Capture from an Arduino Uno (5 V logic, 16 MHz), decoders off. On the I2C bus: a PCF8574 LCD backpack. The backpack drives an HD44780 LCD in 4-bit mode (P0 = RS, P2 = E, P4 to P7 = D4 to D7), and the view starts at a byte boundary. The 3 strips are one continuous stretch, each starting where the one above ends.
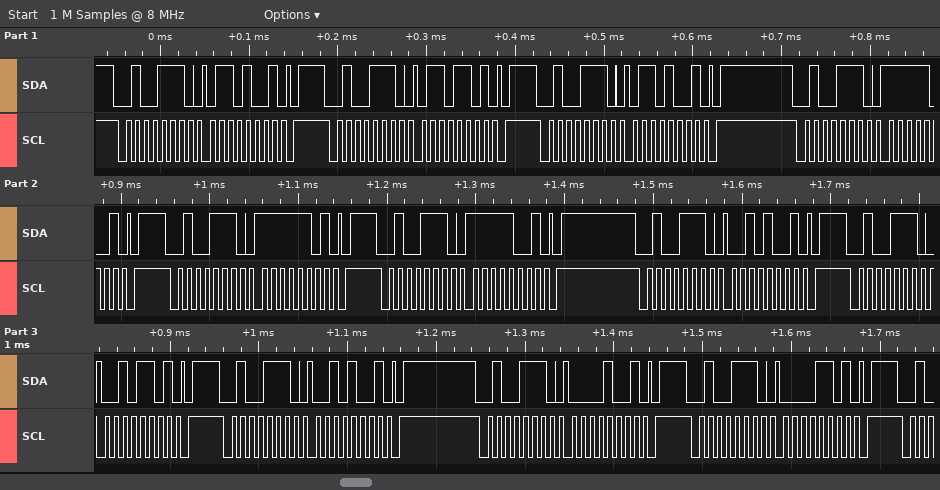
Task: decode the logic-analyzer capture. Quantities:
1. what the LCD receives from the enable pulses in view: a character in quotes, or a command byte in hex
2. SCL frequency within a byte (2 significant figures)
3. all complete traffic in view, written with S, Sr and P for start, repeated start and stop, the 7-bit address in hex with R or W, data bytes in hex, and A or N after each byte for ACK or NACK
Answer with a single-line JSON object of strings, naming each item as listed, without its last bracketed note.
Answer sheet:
{"what the LCD receives from the enable pulses in view: a character in quotes, or a command byte in hex": "'o'", "SCL frequency within a byte": "100 kHz", "all complete traffic in view, written with S, Sr and P for start, repeated start and stop, the 7-bit address in hex with R or W, data bytes in hex, and A or N after each byte for ACK or NACK": "S 27W A 69 A P S 27W A 6D A P S 27W A 69 A P S 27W A F9 A P S 27W A FD A P S 27W A F9 A P S 27W A 29 A P S 27W A 2D A P S 27W A 29 A P S 27W A 09 A P S 27W A 0D A P"}
